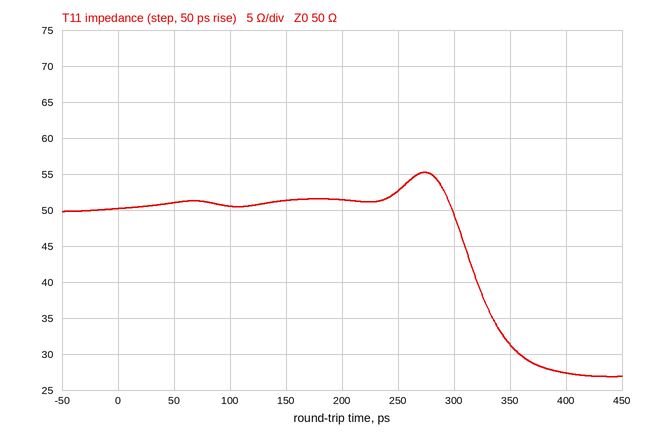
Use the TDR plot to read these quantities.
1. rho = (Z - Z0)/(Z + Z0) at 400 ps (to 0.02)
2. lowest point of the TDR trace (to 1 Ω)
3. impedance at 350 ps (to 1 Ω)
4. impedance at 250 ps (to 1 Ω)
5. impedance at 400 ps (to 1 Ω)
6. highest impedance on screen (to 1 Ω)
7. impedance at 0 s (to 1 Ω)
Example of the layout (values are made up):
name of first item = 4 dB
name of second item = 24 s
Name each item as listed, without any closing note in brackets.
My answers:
rho = (Z - Z0)/(Z + Z0) at 400 ps = -0.30
lowest point of the TDR trace = 27 Ω
impedance at 350 ps = 31 Ω
impedance at 250 ps = 53 Ω
impedance at 400 ps = 27 Ω
highest impedance on screen = 55 Ω
impedance at 0 s = 50 Ω
